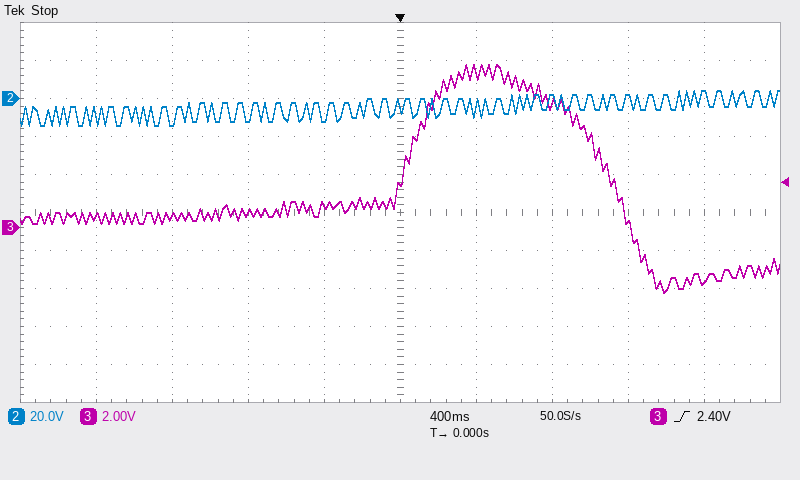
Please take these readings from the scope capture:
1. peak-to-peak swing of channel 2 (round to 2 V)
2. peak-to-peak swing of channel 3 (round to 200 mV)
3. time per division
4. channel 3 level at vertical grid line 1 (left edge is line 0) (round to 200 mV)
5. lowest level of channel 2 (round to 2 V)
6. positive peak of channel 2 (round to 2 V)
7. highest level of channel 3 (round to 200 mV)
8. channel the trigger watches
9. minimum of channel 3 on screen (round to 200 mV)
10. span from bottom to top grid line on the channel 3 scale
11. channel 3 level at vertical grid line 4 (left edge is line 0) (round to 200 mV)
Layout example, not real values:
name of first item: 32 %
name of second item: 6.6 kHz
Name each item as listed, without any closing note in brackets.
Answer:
peak-to-peak swing of channel 2: 18 V
peak-to-peak swing of channel 3: 12.0 V
time per division: 400 ms
channel 3 level at vertical grid line 1 (left edge is line 0): 600 mV
lowest level of channel 2: -14 V
positive peak of channel 2: 4 V
highest level of channel 3: 8.6 V
channel the trigger watches: channel 3
minimum of channel 3 on screen: -3.4 V
span from bottom to top grid line on the channel 3 scale: 20 V
channel 3 level at vertical grid line 4 (left edge is line 0): 1.2 V
